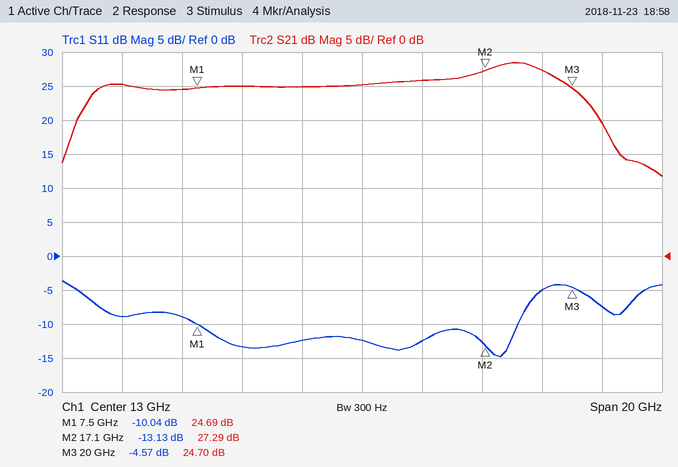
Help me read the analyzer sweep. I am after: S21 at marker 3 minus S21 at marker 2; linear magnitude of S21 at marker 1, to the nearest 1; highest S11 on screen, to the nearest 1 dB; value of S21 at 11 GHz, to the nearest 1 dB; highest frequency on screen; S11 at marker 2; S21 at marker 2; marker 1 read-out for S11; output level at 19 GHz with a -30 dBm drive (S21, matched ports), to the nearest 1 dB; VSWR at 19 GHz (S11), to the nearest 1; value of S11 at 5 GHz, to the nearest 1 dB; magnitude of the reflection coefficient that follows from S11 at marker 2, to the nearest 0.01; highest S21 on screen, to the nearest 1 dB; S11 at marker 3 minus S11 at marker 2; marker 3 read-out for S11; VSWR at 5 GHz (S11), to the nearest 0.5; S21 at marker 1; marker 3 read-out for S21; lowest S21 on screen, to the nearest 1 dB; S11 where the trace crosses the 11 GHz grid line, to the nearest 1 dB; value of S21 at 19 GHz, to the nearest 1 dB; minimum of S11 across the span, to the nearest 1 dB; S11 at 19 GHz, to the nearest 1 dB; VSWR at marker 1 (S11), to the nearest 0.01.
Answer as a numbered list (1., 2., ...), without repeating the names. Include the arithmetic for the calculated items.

1. 24.7 − (27.29) = -2.59 dB
2. 10^(24.69/20) ≈ 17
3. -4 dB
4. 25 dB
5. 23 GHz
6. -13.13 dB
7. 27.29 dB
8. -10.04 dB
9. -30 dBm + (27 dB) = -3 dBm
10. |Γ| = 10^(-5/20) = 0.5623; VSWR = (1 + 0.5623)/(1 − 0.5623) ≈ 4
11. -9 dB
12. 10^(-13.13/20) ≈ 0.22
13. 28 dB
14. -4.57 − (-13.13) = 8.56 dB
15. -4.57 dB
16. |Γ| = 10^(-9/20) = 0.3548; VSWR = (1 + 0.3548)/(1 − 0.3548) ≈ 2.10, so 2.0 to the nearest 0.5
17. 24.69 dB
18. 24.70 dB
19. 12 dB
20. -12 dB
21. 27 dB
22. -15 dB
23. -5 dB
24. (1 + 0.3148)/(1 − 0.3148) ≈ 1.92
